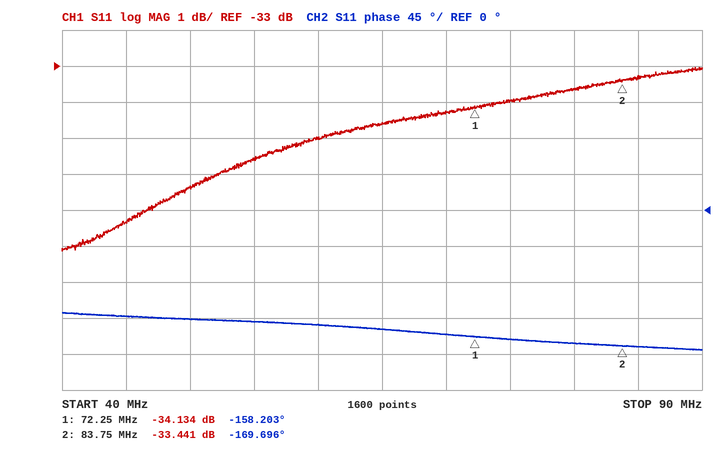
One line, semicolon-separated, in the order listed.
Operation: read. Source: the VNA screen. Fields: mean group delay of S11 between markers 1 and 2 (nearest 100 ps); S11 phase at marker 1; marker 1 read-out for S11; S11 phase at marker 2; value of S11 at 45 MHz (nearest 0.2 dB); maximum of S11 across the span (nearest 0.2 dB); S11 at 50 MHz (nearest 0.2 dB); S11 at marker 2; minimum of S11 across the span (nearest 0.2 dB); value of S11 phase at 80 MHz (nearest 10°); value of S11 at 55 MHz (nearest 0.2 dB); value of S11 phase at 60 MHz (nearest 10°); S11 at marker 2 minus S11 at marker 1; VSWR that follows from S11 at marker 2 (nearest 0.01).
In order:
2.8 ns; -158.203°; -34.134 dB; -169.696°; -37.4 dB; -33.0 dB; -36.4 dB; -33.441 dB; -38.2 dB; -170°; -35.6 dB; -140°; 0.693 dB; 1.04
